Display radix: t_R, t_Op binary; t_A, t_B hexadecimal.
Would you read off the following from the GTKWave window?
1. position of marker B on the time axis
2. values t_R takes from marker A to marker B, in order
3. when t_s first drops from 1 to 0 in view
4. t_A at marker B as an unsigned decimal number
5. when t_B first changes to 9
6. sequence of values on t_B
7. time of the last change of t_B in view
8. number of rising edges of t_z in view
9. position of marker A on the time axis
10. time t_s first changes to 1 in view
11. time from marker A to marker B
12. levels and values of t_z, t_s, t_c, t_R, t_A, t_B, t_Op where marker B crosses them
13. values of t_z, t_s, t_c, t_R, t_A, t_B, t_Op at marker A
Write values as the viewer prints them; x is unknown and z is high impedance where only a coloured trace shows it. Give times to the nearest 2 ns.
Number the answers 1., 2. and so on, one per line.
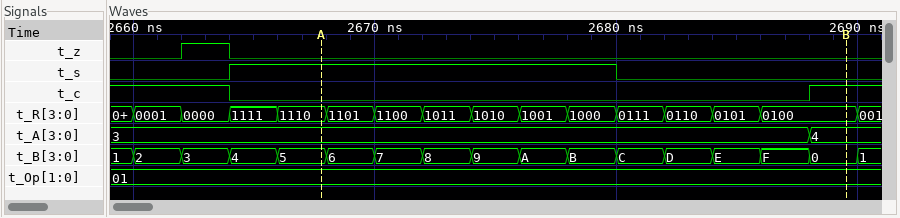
1. 2690 ns
2. 1110, 1101, 1100, 1011, 1010, 1001, 1000, 0111, 0110, 0101, 0100
3. 2680 ns
4. 4
5. 2674 ns
6. 1, 2, 3, 4, 5, 6, 7, 8, 9, A, B, C, D, E, F, 0, 1
7. 2690 ns
8. 1
9. 2668 ns
10. 2664 ns
11. 22 ns
12. t_z=0, t_s=0, t_c=1, t_R=0100, t_A=4, t_B=0, t_Op=01
13. t_z=0, t_s=1, t_c=0, t_R=1110, t_A=3, t_B=5, t_Op=01
